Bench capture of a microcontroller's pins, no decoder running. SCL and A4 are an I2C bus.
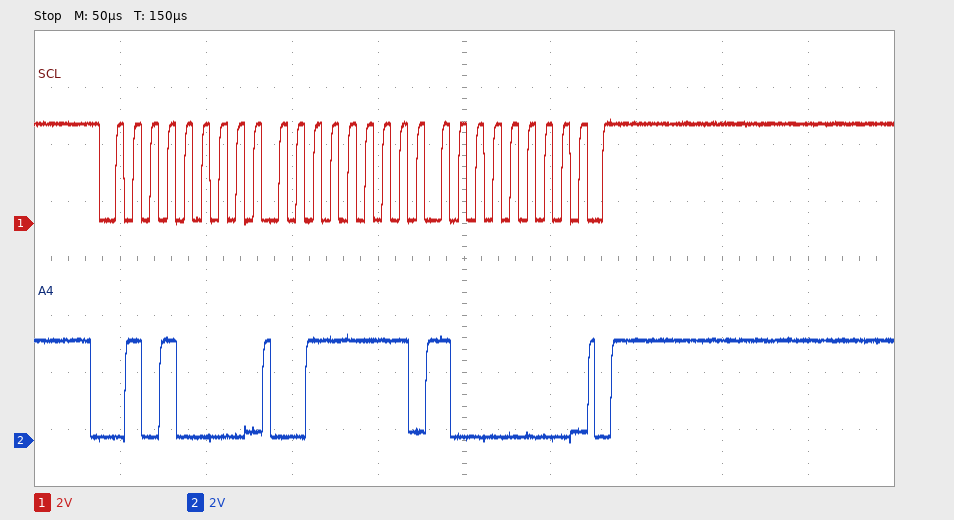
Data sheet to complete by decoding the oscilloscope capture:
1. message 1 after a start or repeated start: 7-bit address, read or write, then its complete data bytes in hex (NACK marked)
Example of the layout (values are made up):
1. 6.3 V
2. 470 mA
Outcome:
1. 0x28 write: 3F 80
